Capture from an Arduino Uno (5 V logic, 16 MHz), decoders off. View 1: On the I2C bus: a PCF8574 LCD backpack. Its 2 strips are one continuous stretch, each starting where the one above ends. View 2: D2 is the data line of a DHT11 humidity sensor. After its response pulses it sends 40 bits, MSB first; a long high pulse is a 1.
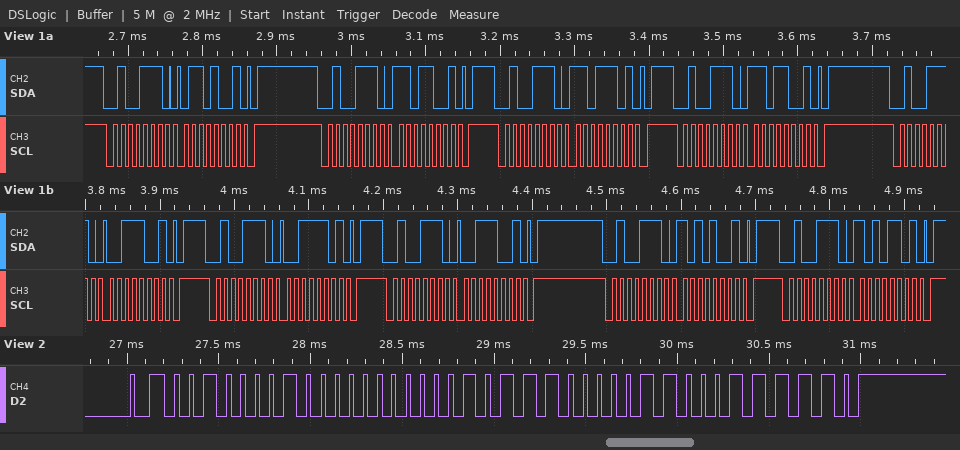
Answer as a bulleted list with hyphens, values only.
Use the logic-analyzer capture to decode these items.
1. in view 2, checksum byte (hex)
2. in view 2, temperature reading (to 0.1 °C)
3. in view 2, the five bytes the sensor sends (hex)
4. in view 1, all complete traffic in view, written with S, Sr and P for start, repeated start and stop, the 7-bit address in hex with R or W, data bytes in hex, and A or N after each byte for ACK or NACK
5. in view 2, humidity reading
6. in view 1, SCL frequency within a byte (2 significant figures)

- 0x3E
- 23.6 °C
- 21 00 17 06 3E
- S 27W A 69 A P S 27W A D9 A P S 27W A DD A P S 27W A D9 A P S 27W A 39 A P S 27W A 3D A P S 27W A 39 A P S 27W A A9 A P S 27W A AD A P
- 33 %
- 100 kHz
